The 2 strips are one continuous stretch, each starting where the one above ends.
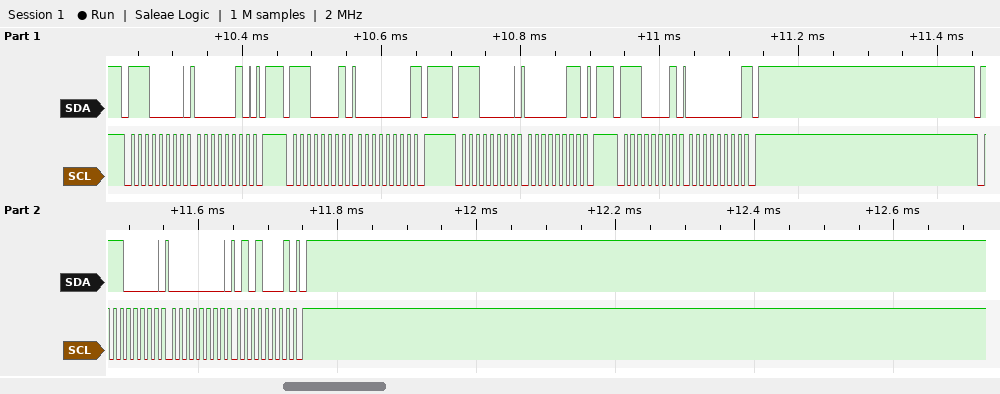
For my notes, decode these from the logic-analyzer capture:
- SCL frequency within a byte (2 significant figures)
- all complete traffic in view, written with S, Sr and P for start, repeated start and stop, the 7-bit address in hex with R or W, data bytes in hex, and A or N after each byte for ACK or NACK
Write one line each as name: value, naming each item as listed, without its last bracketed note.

SCL frequency within a byte: 100 kHz
all complete traffic in view, written with S, Sr and P for start, repeated start and stop, the 7-bit address in hex with R or W, data bytes in hex, and A or N after each byte for ACK or NACK: S 70W A 02 A P S 70R A 00 N P S 70W A 03 A P S 70R A 00 N P S 70W A 00 A 51 A P
